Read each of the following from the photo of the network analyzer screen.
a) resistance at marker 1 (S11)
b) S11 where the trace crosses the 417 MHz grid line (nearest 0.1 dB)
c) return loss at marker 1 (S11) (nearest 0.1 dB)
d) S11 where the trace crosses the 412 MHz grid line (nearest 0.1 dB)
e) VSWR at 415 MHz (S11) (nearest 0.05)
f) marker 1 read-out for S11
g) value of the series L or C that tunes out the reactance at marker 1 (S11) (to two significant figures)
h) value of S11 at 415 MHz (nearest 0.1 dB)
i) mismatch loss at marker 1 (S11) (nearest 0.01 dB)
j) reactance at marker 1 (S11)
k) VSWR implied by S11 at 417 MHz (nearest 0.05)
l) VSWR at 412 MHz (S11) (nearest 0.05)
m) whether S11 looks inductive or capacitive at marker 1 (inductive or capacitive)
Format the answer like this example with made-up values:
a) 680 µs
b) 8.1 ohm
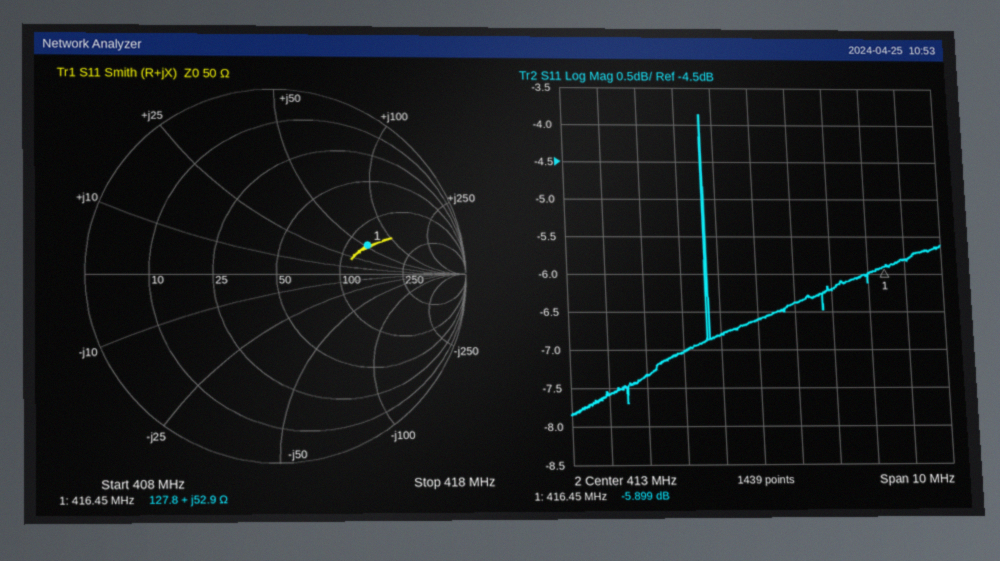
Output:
a) 127.8 Ω
b) -5.8 dB
c) 5.9 dB
d) -6.8 dB
e) 2.90
f) -5.899 dB
g) 7.2 pF
h) -6.2 dB
i) 1.29 dB
j) +52.9 Ω
k) 3.10
l) 2.70
m) inductive
